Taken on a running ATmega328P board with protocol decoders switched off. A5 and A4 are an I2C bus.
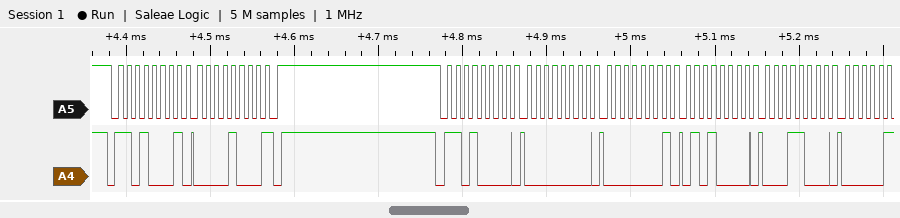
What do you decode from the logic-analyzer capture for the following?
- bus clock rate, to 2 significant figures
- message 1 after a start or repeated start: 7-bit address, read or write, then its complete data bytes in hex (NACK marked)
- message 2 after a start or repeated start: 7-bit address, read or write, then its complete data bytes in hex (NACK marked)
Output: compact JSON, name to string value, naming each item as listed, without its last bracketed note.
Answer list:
{"bus clock rate, to 2 significant figures": "100 kHz", "message 1 after a start or repeated start: 7-bit address, read or write, then its complete data bytes in hex": "0x68 read: 08 NACK", "message 2 after a start or repeated start: 7-bit address, read or write, then its complete data bytes in hex": "0x68 write: 00 01 50 18"}
